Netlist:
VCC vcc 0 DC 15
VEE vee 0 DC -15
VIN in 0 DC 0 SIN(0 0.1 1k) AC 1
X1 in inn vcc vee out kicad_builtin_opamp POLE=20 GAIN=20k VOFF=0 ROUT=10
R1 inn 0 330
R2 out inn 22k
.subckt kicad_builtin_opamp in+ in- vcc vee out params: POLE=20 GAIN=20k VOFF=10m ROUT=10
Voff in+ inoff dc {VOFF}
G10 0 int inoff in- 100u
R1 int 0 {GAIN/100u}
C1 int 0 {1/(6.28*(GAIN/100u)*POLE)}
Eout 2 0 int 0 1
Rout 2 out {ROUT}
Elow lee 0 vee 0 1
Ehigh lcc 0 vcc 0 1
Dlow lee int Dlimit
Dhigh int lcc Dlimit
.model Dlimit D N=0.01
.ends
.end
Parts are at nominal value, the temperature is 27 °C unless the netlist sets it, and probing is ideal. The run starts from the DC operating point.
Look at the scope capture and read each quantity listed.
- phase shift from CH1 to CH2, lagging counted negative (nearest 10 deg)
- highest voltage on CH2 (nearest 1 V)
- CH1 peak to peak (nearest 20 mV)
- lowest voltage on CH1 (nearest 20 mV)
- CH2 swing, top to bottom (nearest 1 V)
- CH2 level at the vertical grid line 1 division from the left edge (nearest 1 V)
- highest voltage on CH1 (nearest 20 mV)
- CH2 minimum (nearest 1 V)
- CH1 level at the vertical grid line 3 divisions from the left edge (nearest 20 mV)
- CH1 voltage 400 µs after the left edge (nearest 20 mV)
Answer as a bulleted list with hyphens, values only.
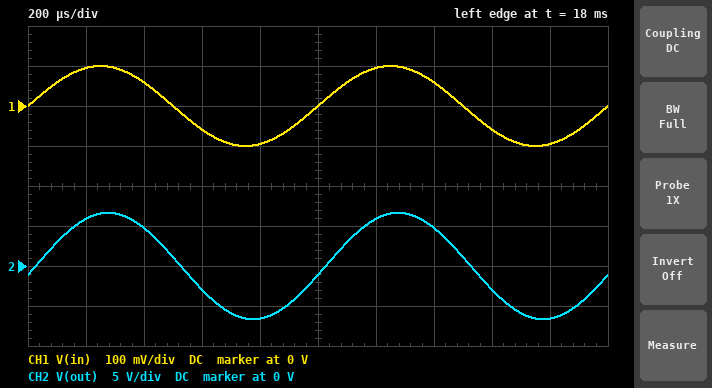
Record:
- -10 deg
- 7 V
- 200 mV
- -100 mV
- 13 V
- 6 V
- 100 mV
- -7 V
- -60 mV
- 60 mV
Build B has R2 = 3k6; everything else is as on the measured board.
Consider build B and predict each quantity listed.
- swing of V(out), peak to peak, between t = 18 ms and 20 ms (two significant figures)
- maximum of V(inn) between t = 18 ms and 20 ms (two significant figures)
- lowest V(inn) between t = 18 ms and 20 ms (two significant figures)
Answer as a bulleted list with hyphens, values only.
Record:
- 2.4 V
- 100 mV
- -100 mV
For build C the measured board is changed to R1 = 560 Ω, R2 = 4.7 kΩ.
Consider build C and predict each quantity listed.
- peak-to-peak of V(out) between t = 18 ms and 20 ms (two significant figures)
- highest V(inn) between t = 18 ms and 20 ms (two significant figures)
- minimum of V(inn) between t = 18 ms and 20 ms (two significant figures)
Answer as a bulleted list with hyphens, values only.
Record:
- 1.9 V
- 100 mV
- -100 mV
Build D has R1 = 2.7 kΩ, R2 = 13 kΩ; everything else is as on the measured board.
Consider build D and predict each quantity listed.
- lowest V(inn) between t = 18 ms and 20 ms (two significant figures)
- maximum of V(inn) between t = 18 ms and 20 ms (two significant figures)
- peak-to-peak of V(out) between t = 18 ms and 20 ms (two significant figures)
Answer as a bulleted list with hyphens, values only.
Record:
- -100 mV
- 100 mV
- 1.2 V
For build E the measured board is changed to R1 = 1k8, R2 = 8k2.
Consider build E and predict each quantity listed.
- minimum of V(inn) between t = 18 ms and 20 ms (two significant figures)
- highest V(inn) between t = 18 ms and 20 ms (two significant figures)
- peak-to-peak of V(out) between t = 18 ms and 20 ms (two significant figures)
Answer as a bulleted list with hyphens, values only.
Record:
- -100 mV
- 100 mV
- 1.1 V
